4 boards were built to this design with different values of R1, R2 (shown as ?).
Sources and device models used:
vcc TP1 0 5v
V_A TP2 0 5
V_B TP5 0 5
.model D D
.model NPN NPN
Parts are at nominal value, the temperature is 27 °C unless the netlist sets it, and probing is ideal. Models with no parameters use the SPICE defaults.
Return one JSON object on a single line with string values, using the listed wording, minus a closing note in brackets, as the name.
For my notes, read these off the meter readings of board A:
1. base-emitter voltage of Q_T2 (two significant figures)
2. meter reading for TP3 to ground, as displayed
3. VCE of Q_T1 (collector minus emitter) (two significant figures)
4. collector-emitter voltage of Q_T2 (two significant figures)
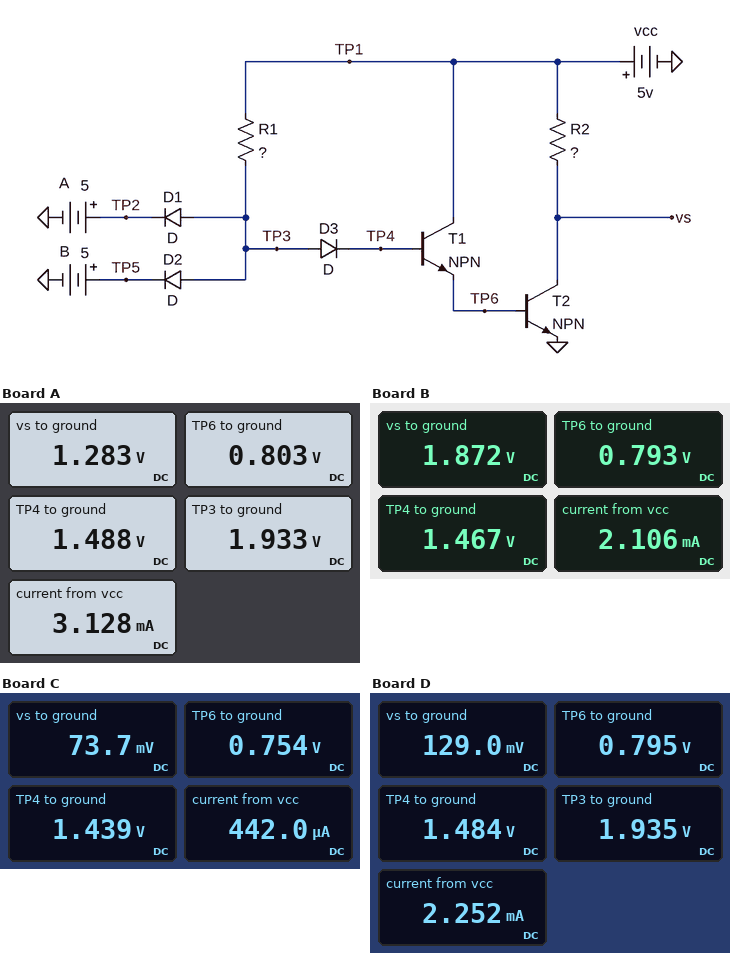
{"base-emitter voltage of Q_T2": "800 mV", "meter reading for TP3 to ground, as displayed": "1.933 V", "VCE of Q_T1 (collector minus emitter)": "4.2 V", "collector-emitter voltage of Q_T2": "1.3 V"}
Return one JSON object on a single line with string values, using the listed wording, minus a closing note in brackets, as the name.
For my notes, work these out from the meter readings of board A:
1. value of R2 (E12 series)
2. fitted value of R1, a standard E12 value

{"value of R2": "1.2 kΩ", "fitted value of R1, a standard E12 value": "10 MΩ"}
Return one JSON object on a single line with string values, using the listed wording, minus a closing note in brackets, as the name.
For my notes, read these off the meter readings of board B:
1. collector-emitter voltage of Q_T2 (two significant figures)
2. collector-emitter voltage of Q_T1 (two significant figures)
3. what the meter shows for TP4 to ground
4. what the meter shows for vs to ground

{"collector-emitter voltage of Q_T2": "1.9 V", "collector-emitter voltage of Q_T1": "4.2 V", "what the meter shows for TP4 to ground": "1.467 V", "what the meter shows for vs to ground": "1.872 V"}
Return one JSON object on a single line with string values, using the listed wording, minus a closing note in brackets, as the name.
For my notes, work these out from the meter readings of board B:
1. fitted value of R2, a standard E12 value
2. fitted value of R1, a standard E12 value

{"fitted value of R2, a standard E12 value": "1.5 kΩ", "fitted value of R1, a standard E12 value": "15 MΩ"}
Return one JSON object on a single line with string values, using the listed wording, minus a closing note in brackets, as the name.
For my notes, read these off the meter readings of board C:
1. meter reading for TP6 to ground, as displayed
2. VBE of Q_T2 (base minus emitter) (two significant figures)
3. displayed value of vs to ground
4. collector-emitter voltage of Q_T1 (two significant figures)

{"meter reading for TP6 to ground, as displayed": "0.754 V", "VBE of Q_T2 (base minus emitter)": "750 mV", "displayed value of vs to ground": "73.7 mV", "collector-emitter voltage of Q_T1": "4.2 V"}
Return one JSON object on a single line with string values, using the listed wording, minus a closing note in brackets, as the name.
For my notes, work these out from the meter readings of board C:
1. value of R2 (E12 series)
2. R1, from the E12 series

{"value of R2": "12 kΩ", "R1, from the E12 series": "10 MΩ"}
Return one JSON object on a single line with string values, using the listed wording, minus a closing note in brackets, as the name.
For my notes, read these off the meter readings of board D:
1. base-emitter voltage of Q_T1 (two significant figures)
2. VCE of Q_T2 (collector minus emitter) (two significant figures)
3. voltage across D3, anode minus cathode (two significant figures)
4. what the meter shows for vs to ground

{"base-emitter voltage of Q_T1": "690 mV", "VCE of Q_T2 (collector minus emitter)": "130 mV", "voltage across D3, anode minus cathode": "450 mV", "what the meter shows for vs to ground": "129.0 mV"}
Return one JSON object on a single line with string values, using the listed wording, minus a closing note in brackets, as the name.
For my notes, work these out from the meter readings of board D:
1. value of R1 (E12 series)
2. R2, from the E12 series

{"value of R1": "8.2 MΩ", "R2, from the E12 series": "2.2 kΩ"}
